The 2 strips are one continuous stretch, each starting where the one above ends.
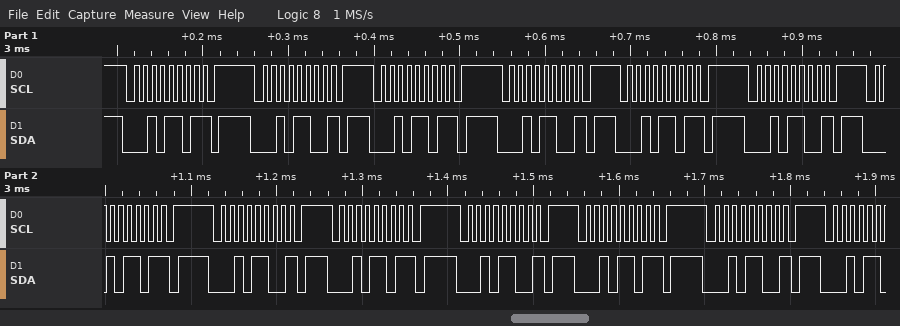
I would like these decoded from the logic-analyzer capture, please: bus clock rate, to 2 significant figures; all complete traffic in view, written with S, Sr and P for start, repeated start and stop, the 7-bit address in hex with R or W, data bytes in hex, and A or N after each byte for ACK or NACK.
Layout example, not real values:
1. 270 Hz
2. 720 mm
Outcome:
1. 100 kHz
2. S 16R N P S 16W N P S 16R N P S 16W N P S 16R N P S 16W N P S 16R N P S 16W N P S 16R N P S 16W N P S 16R N P S 16W N P
